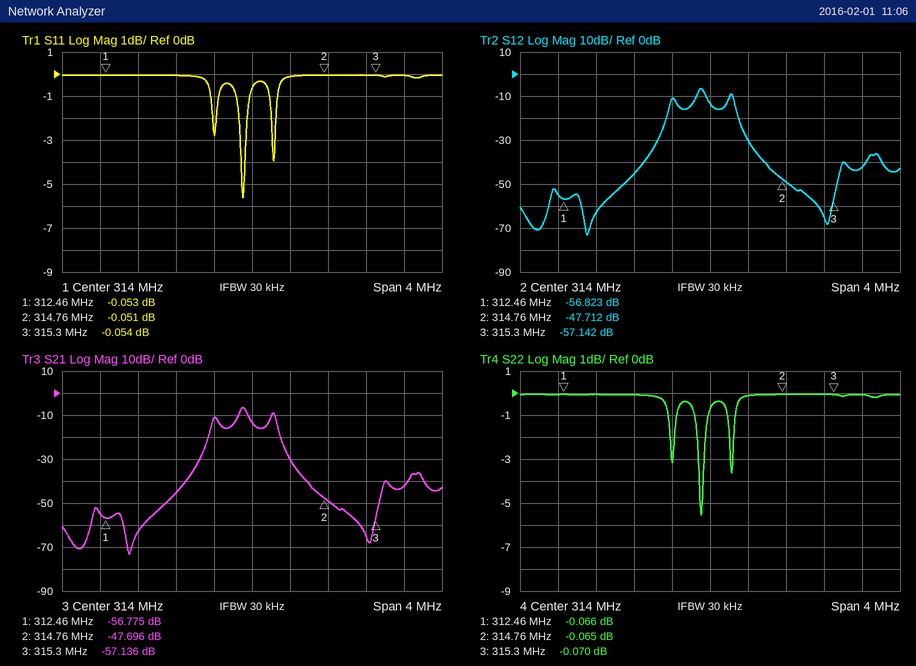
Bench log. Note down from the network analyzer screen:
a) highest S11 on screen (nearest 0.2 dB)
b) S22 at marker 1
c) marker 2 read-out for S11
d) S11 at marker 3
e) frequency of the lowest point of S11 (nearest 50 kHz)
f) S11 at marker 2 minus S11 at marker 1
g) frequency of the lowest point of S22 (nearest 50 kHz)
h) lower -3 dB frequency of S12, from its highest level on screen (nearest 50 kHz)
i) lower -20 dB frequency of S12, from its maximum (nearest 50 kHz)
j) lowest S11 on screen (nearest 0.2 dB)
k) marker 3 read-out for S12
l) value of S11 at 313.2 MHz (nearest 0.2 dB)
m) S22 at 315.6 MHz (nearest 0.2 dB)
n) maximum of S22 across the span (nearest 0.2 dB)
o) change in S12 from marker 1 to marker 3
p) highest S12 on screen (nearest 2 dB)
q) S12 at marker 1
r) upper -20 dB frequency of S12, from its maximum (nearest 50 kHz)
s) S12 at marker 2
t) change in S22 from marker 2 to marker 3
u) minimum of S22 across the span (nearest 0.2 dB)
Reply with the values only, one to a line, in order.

0.0 dB
-0.066 dB
-0.051 dB
-0.054 dB
313.90 MHz
0.002 dB
313.90 MHz
313.85 MHz
313.50 MHz
-5.6 dB
-57.142 dB
0.0 dB
0.0 dB
0.0 dB
-0.319 dB
-6 dB
-56.823 dB
314.35 MHz
-47.712 dB
-0.005 dB
-5.6 dB
